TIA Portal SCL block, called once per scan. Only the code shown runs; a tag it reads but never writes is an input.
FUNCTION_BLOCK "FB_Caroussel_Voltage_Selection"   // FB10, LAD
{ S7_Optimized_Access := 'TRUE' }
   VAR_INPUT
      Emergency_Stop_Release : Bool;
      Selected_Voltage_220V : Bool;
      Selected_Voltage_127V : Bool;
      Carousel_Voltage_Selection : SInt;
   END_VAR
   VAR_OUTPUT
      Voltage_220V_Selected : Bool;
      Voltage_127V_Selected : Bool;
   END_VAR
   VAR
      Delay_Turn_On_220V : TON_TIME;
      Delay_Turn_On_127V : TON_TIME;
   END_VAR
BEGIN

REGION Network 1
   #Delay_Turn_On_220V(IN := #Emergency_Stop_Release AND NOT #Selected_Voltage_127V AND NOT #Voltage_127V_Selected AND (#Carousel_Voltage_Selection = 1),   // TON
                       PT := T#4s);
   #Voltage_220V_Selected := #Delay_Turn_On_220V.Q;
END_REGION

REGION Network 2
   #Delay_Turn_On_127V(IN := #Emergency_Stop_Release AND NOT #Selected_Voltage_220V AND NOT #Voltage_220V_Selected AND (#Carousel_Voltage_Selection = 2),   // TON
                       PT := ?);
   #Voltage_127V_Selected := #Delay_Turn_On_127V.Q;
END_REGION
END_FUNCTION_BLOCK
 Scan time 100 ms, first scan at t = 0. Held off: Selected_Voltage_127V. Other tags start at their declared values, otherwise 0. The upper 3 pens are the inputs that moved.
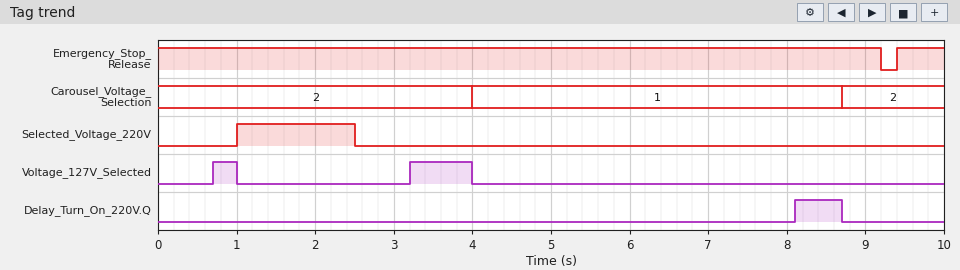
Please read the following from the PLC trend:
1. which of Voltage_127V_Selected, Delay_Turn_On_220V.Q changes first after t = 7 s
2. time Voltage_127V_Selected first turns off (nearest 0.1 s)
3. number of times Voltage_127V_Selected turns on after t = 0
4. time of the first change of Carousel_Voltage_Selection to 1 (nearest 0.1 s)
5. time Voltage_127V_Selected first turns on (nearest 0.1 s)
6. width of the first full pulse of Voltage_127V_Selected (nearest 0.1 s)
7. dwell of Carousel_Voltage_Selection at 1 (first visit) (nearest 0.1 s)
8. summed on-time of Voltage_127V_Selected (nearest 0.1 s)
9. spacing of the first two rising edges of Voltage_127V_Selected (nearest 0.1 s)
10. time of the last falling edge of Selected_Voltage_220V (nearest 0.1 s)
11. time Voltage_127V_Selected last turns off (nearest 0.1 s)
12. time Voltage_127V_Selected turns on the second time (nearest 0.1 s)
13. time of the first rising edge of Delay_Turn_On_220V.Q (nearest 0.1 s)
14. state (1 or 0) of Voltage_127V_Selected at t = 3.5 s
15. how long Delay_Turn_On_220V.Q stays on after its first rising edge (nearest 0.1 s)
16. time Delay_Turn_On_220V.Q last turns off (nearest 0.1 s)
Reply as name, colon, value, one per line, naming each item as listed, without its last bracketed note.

which of Voltage_127V_Selected, Delay_Turn_On_220V.Q changes first after t = 7 s: Delay_Turn_On_220V.Q
time Voltage_127V_Selected first turns off: 1.0 s
number of times Voltage_127V_Selected turns on after t = 0: 2
time of the first change of Carousel_Voltage_Selection to 1: 4.0 s
time Voltage_127V_Selected first turns on: 0.7 s
width of the first full pulse of Voltage_127V_Selected: 0.3 s
dwell of Carousel_Voltage_Selection at 1 (first visit): 4.7 s
summed on-time of Voltage_127V_Selected: 1.1 s
spacing of the first two rising edges of Voltage_127V_Selected: 2.5 s
time of the last falling edge of Selected_Voltage_220V: 2.5 s
time Voltage_127V_Selected last turns off: 4.0 s
time Voltage_127V_Selected turns on the second time: 3.2 s
time of the first rising edge of Delay_Turn_On_220V.Q: 8.1 s
state (1 or 0) of Voltage_127V_Selected at t = 3.5 s: 1
how long Delay_Turn_On_220V.Q stays on after its first rising edge: 0.6 s
time Delay_Turn_On_220V.Q last turns off: 8.7 s
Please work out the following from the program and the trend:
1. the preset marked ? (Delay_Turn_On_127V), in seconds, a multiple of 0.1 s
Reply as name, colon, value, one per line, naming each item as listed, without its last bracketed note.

the preset marked ? (Delay_Turn_On_127V), in seconds, a multiple of 0.1 s: 0.7 s
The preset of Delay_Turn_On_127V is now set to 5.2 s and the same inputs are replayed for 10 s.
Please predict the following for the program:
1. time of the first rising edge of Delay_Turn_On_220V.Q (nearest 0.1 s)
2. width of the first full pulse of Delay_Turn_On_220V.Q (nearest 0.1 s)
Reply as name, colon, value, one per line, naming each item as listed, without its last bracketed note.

time of the first rising edge of Delay_Turn_On_220V.Q: 8.0 s
width of the first full pulse of Delay_Turn_On_220V.Q: 0.7 s
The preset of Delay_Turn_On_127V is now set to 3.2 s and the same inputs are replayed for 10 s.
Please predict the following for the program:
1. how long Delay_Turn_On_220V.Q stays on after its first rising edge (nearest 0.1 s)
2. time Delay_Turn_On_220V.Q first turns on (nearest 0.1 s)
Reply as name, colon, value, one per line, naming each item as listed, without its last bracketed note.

how long Delay_Turn_On_220V.Q stays on after its first rising edge: 0.7 s
time Delay_Turn_On_220V.Q first turns on: 8.0 s
